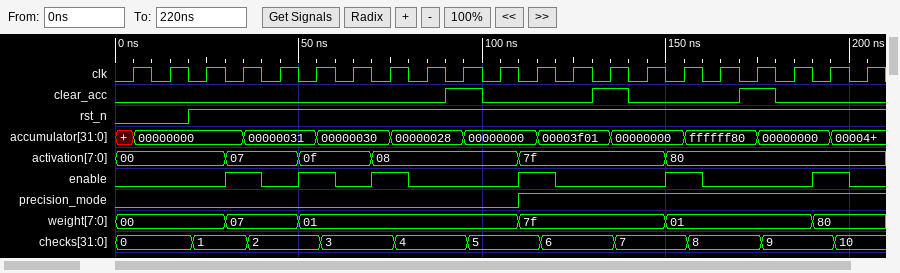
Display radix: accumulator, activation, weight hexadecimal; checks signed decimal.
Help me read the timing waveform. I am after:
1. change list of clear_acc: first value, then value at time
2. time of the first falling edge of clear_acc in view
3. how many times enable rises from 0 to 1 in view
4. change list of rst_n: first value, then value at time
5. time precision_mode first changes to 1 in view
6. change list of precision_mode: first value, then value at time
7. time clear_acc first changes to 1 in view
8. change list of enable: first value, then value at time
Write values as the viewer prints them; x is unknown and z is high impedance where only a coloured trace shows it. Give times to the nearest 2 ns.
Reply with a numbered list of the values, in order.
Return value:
1. 0, 1 at 90 ns, 0 at 100 ns, 1 at 130 ns, 0 at 140 ns, 1 at 170 ns, 0 at 180 ns
2. 100 ns
3. 6
4. 0, 1 at 20 ns
5. 110 ns
6. 0, 1 at 110 ns
7. 90 ns
8. 0, 1 at 30 ns, 0 at 40 ns, 1 at 50 ns, 0 at 60 ns, 1 at 70 ns, 0 at 80 ns, 1 at 110 ns, 0 at 120 ns, 1 at 150 ns, 0 at 160 ns, 1 at 190 ns, 0 at 200 ns
